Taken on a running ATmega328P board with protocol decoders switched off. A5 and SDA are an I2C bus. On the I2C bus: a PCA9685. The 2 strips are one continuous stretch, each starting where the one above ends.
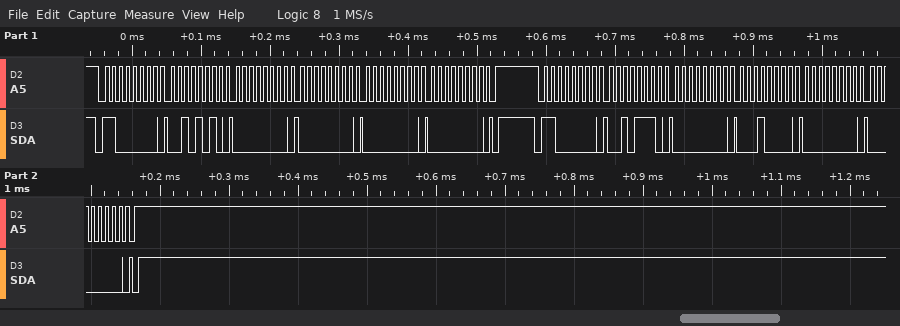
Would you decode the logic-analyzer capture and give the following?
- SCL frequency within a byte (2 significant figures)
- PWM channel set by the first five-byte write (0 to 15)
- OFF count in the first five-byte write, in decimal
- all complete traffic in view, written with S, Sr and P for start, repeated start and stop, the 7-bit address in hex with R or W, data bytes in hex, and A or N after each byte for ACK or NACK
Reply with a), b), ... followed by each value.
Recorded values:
a) 100 kHz
b) 9
c) 0
d) S 60W A 2A A 00 A 00 A 00 A 00 A P S 60W A 2E A 00 A 10 A 00 A 00 A P
